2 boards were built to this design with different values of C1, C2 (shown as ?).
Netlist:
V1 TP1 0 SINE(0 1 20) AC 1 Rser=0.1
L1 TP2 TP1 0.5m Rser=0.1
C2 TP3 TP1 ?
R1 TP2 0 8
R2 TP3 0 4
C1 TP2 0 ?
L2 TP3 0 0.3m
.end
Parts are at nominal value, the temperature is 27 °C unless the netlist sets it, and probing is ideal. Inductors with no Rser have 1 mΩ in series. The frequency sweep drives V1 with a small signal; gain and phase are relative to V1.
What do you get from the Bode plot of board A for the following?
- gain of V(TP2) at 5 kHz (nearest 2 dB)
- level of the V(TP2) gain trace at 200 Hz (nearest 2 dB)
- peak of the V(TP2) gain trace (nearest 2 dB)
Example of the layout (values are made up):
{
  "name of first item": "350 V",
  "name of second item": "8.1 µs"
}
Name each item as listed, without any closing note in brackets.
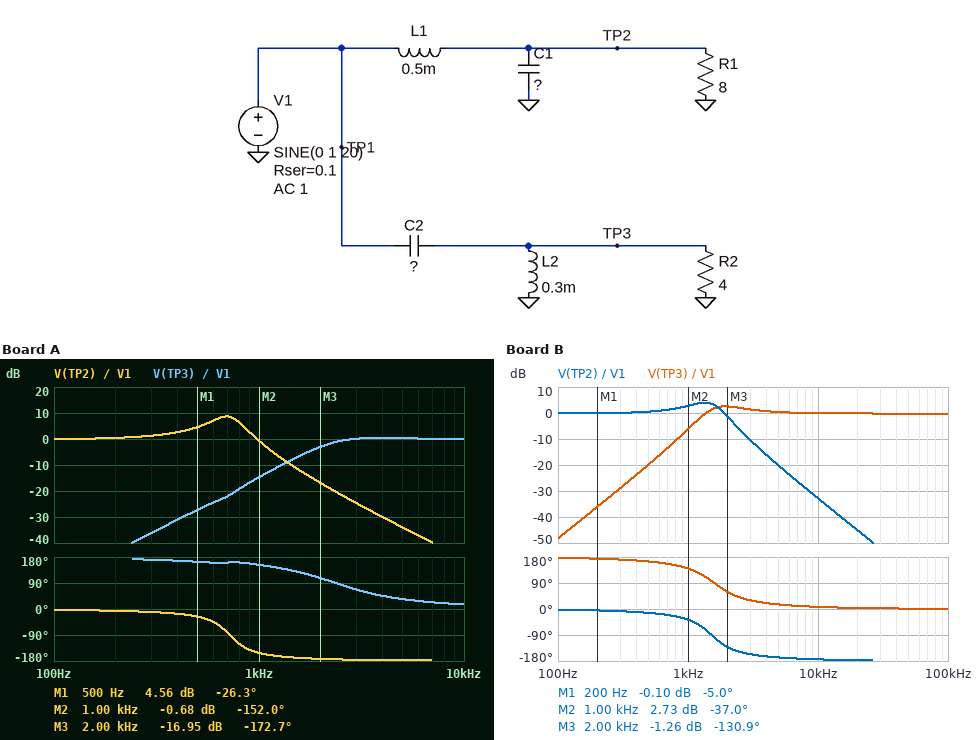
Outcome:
{
  "gain of V(TP2) at 5 kHz": "-34 dB",
  "level of the V(TP2) gain trace at 200 Hz": "0 dB",
  "peak of the V(TP2) gain trace": "8 dB"
}
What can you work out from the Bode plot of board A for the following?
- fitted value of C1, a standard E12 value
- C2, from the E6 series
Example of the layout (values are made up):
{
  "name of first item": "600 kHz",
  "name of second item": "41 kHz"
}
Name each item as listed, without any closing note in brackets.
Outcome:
{
  "fitted value of C1, a standard E12 value": "100 µF",
  "C2, from the E6 series": "15 µF"
}
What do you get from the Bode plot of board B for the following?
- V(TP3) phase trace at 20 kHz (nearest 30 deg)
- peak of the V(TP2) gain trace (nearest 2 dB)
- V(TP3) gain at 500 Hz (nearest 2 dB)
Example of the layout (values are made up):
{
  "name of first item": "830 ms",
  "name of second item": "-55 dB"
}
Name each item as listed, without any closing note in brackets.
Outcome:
{
  "V(TP3) phase trace at 20 kHz": "0 deg",
  "peak of the V(TP2) gain trace": "4 dB",
  "V(TP3) gain at 500 Hz": "-20 dB"
}
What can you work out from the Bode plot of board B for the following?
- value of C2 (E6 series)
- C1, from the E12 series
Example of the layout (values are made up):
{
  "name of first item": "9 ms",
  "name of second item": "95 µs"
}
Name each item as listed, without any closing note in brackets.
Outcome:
{
  "value of C2": "33 µF",
  "C1, from the E12 series": "22 µF"
}
